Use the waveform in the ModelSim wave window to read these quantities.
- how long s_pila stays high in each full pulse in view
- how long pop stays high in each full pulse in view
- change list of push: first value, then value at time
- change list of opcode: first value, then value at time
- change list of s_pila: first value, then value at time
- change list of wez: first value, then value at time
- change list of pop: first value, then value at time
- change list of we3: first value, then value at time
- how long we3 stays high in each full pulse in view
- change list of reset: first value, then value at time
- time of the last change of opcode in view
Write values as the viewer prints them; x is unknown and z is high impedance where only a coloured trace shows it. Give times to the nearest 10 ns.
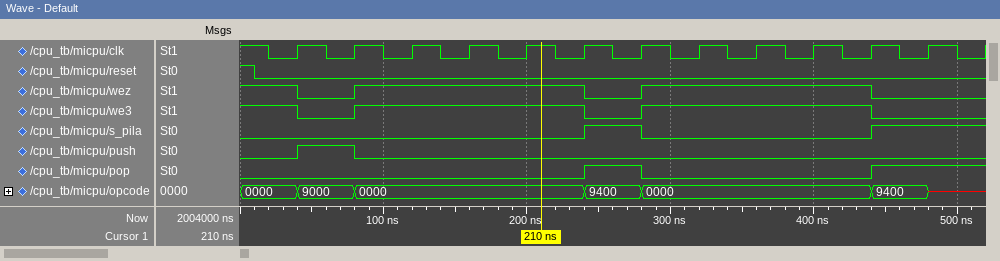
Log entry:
40 ns
40 ns
0, 1 at 40 ns, 0 at 80 ns
0000, 9000 at 40 ns, 0000 at 80 ns, 9400 at 240 ns, 0000 at 280 ns, 9400 at 440 ns, x at 480 ns
0, 1 at 240 ns, 0 at 280 ns, 1 at 440 ns
1, 0 at 40 ns, 1 at 80 ns, 0 at 240 ns, 1 at 280 ns, 0 at 440 ns
0, 1 at 240 ns, 0 at 280 ns, 1 at 440 ns
1, 0 at 40 ns, 1 at 80 ns, 0 at 240 ns, 1 at 280 ns, 0 at 440 ns
160 ns, 160 ns
1, 0 at 10 ns
480 ns
